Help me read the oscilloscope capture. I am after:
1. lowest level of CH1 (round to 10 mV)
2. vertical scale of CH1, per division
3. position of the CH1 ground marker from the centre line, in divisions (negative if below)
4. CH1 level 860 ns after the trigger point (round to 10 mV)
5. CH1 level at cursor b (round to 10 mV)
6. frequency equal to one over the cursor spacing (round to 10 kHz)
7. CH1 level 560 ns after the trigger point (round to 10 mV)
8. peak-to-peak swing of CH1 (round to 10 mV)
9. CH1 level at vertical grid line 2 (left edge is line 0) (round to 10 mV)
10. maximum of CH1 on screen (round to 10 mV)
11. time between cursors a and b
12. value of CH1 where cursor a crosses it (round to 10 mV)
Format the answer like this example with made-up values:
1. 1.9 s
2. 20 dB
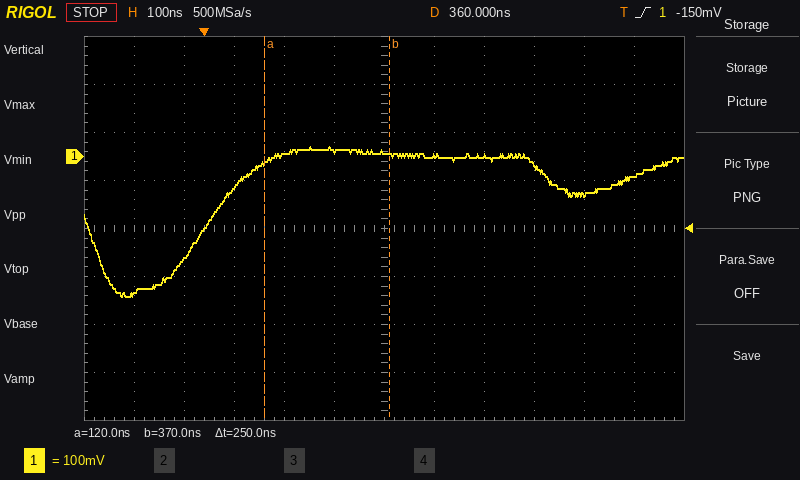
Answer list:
1. -290 mV
2. 100 mV
3. +1.5 div
4. -40 mV
5. 0 mV
6. 4.00 MHz
7. 0 mV
8. 310 mV
9. -210 mV
10. 20 mV
11. 250 ns
12. -10 mV
